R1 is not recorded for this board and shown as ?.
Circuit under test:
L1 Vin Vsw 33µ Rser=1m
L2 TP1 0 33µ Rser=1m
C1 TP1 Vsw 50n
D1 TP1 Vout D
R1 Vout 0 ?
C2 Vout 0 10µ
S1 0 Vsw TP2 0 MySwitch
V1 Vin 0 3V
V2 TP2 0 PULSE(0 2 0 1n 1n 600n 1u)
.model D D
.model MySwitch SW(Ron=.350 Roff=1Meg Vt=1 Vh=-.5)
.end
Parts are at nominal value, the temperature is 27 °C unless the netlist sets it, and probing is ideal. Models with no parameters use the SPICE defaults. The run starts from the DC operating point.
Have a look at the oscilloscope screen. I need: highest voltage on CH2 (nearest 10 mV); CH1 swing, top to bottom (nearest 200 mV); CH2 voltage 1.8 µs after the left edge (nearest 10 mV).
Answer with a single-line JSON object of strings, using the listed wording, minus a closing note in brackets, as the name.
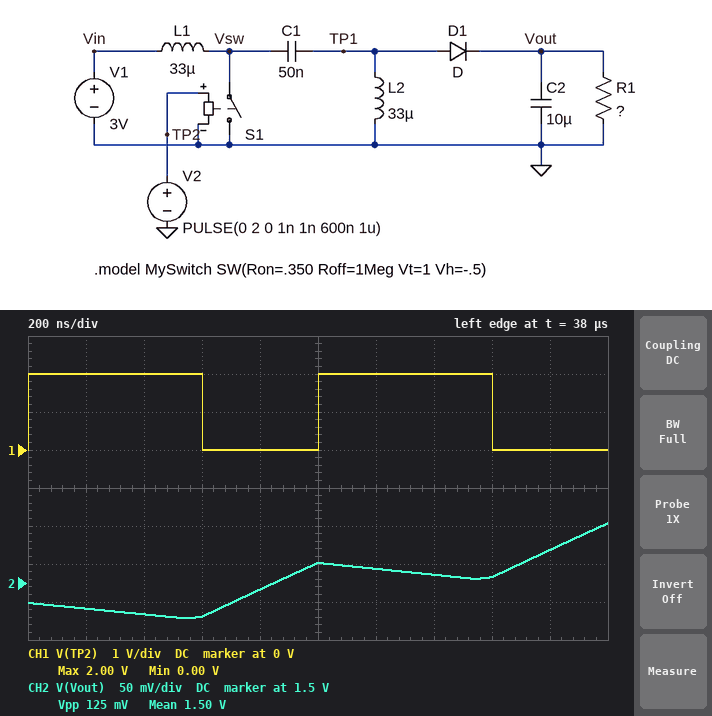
{"highest voltage on CH2": "1.58 V", "CH1 swing, top to bottom": "2.0 V", "CH2 voltage 1.8 µs after the left edge": "1.54 V"}
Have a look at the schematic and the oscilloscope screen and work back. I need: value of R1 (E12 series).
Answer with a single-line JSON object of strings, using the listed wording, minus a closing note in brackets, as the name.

{"value of R1": "3.9 Ω"}
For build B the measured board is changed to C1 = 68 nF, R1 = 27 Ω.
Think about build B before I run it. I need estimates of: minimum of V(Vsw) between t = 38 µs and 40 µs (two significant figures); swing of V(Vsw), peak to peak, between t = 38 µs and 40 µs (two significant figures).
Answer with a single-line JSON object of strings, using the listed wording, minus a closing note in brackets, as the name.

{"minimum of V(Vsw) between t = 38 µs and 40 µs": "710 mV", "swing of V(Vsw), peak to peak, between t = 38 µs and 40 µs": "9.2 V"}
